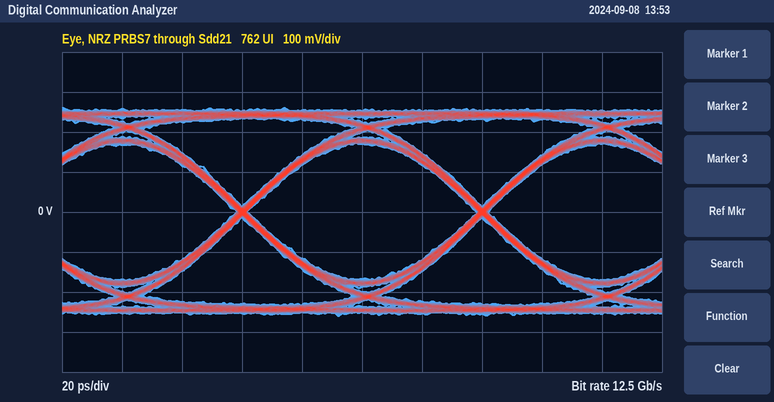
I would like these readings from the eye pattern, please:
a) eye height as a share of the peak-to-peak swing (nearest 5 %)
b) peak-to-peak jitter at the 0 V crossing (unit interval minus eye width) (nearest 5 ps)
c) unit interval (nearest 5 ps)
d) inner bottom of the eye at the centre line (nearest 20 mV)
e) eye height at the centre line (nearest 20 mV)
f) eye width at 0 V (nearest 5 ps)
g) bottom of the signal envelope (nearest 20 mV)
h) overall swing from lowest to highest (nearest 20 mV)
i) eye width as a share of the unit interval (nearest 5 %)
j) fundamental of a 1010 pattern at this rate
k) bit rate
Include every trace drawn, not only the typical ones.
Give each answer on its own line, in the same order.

65 %
5 ps
80 ps
-160 mV
340 mV
75 ps
-260 mV
520 mV
95 %
6.25 GHz
12.5 Gb/s
